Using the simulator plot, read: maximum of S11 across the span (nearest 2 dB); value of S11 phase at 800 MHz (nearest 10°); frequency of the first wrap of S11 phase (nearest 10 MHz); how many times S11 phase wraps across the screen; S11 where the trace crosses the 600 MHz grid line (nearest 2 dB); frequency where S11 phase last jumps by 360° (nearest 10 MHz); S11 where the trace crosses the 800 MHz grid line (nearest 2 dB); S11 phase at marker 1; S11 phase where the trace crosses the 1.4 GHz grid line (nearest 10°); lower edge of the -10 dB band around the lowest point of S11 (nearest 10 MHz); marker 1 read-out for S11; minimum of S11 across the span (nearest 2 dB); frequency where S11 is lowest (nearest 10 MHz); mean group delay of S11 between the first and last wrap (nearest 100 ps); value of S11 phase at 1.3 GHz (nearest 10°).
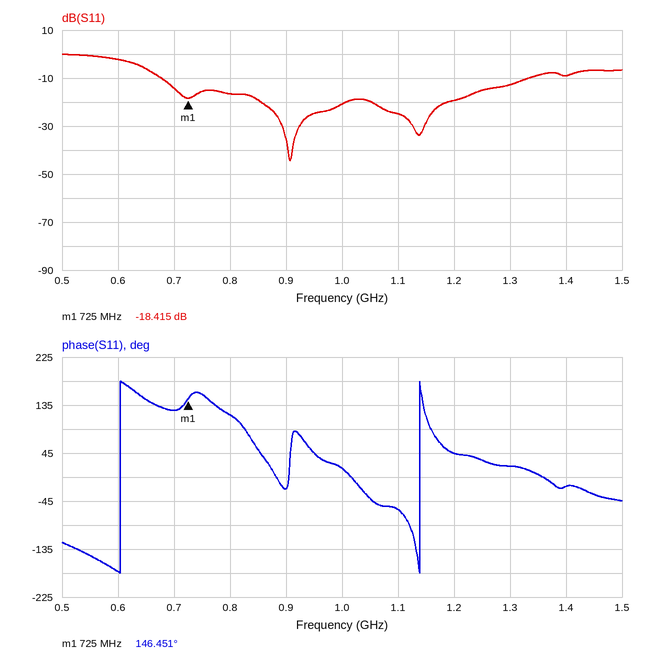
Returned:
0 dB
120°
600 MHz
2
-2 dB
1.14 GHz
-16 dB
146.451°
-20°
680 MHz
-18.415 dB
-44 dB
910 MHz
1.9 ns
20°
